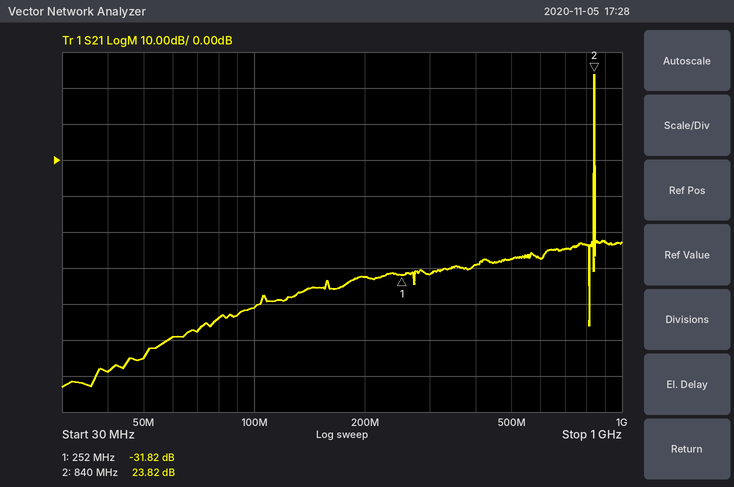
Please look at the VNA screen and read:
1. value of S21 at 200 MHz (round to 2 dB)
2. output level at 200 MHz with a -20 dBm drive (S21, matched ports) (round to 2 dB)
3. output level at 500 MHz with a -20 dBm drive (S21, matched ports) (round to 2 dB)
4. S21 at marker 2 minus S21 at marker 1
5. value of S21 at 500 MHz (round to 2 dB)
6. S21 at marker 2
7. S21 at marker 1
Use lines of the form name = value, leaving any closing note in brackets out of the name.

value of S21 at 200 MHz = -32 dB
output level at 200 MHz with a -20 dBm drive (S21, matched ports) = -52 dBm
output level at 500 MHz with a -20 dBm drive (S21, matched ports) = -48 dBm
S21 at marker 2 minus S21 at marker 1 = 55.64 dB
value of S21 at 500 MHz = -28 dB
S21 at marker 2 = 23.82 dB
S21 at marker 1 = -31.82 dB
